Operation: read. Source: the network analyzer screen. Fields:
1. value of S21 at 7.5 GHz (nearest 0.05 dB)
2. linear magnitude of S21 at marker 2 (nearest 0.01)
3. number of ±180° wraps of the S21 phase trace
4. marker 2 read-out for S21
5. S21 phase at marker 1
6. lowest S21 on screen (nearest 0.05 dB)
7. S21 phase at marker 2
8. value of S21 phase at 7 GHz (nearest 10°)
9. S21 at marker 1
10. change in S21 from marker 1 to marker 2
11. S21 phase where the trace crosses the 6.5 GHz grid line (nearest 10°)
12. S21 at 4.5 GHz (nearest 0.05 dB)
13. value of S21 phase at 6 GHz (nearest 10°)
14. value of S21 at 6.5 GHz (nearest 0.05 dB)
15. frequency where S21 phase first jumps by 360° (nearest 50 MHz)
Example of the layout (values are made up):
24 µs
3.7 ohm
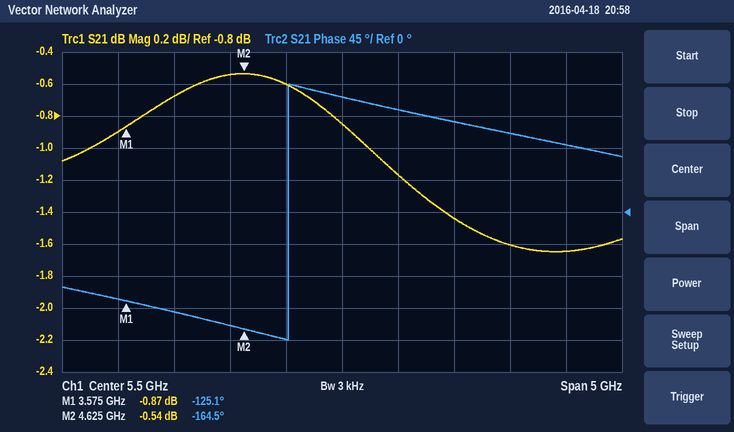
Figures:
-1.65 dB
0.94
1
-0.54 dB
-125.1°
-1.65 dB
-164.5°
110°
-0.87 dB
0.33 dB
130°
-0.55 dB
140°
-1.45 dB
5.00 GHz
